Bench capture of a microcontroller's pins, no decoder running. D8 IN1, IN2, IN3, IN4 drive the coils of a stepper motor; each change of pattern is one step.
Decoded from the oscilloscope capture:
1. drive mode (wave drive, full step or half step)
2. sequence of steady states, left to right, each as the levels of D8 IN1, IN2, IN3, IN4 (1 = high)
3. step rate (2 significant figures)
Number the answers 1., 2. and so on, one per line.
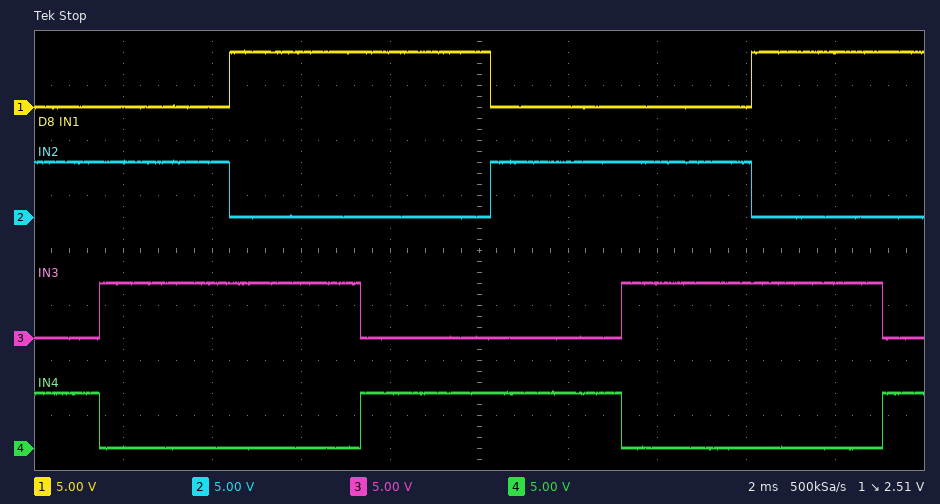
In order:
1. full step
2. 0101 0110 1010 1001 0101 0110 1010 1001
3. 340 steps/s
